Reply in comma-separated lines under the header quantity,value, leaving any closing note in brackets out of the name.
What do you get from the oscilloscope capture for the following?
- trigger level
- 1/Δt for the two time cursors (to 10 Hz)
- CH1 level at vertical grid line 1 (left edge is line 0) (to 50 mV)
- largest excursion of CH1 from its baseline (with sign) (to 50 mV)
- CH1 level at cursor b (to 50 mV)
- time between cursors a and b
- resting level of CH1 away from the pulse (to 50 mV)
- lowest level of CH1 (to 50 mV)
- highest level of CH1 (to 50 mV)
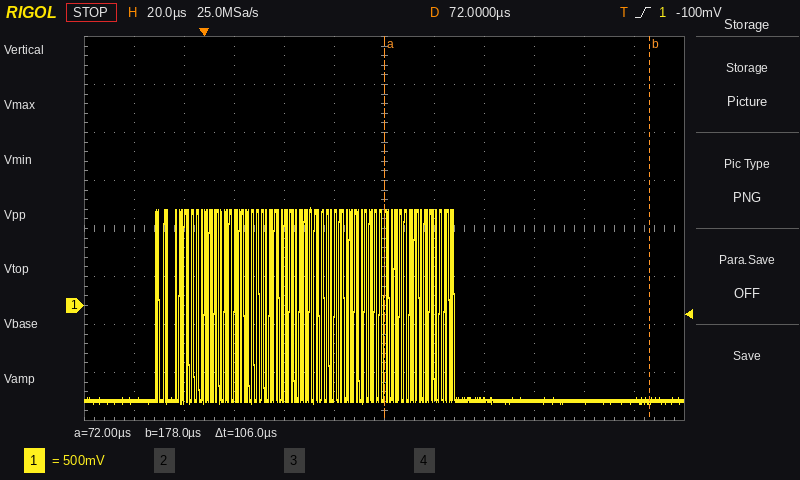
quantity,value
trigger level,-100 mV
1/Δt for the two time cursors,9.43 kHz
CH1 level at vertical grid line 1 (left edge is line 0),-1.00 V
largest excursion of CH1 from its baseline (with sign),+2.00 V
CH1 level at cursor b,-1.00 V
time between cursors a and b,106 µs
resting level of CH1 away from the pulse,-1.00 V
lowest level of CH1,-1.00 V
highest level of CH1,1.00 V
